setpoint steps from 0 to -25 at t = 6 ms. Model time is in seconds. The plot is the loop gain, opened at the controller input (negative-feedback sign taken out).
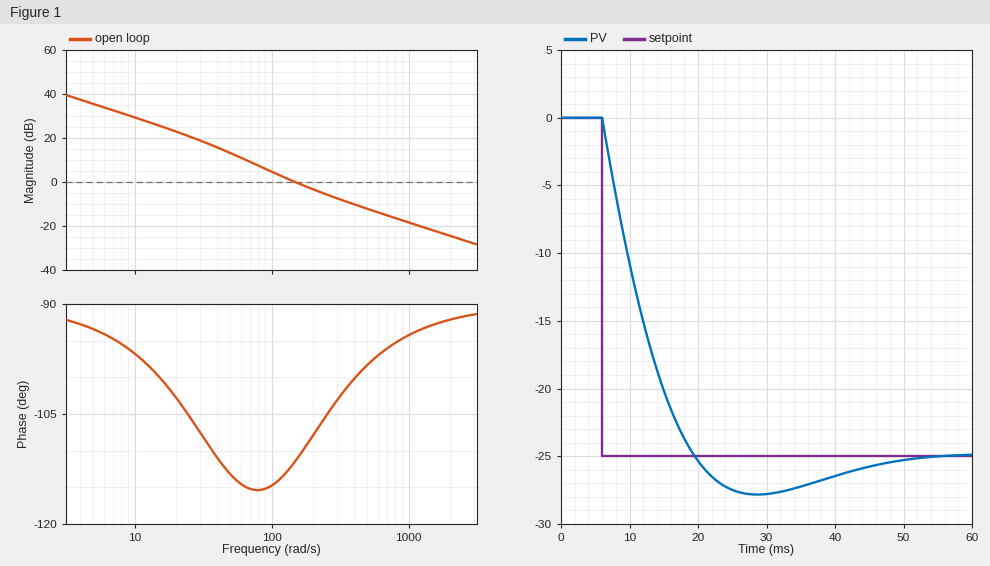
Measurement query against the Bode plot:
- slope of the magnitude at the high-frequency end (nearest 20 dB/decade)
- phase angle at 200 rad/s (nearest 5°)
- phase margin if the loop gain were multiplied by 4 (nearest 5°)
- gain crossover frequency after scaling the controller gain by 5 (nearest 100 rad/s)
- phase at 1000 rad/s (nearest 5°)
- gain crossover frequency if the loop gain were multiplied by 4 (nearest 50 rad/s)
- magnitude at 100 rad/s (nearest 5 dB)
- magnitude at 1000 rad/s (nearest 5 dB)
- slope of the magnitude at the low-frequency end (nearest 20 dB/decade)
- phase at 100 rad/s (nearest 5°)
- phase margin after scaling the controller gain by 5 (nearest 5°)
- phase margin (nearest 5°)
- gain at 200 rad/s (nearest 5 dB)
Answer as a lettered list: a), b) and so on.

a) -20 dB/decade
b) -110°
c) 80°
d) 600 rad/s
e) -95°
f) 500 rad/s
g) 5 dB
h) -20 dB
i) -20 dB/decade
j) -115°
k) 85°
l) 70°
m) -5 dB
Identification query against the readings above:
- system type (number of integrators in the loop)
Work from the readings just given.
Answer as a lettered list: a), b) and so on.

a) 1
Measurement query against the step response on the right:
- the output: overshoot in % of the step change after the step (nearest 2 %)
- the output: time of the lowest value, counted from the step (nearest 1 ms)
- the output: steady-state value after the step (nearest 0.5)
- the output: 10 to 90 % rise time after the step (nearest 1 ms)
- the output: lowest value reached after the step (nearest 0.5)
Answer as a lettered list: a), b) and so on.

a) 12 %
b) 23 ms
c) -25.0
d) 10 ms
e) -28.0
